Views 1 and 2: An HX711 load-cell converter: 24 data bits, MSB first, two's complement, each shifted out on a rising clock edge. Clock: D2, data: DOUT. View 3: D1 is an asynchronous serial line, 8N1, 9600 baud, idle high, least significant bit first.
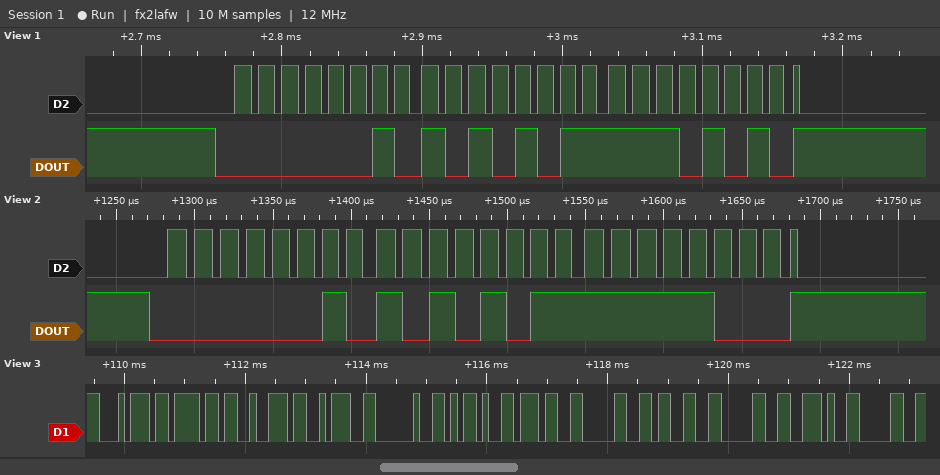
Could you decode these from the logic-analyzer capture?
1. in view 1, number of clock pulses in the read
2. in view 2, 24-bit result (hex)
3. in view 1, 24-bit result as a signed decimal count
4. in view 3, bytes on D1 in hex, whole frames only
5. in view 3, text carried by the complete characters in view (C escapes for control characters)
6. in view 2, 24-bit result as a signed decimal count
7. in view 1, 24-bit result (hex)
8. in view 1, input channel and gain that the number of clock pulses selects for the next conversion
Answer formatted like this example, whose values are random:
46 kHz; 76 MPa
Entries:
25; 0x02ABF8; 175082; 74 6F 72 3A 20 2D 37 30 33 30 2E 30; "tor: -7030.0"; 175096; 0x02ABEA; channel A, gain 128
